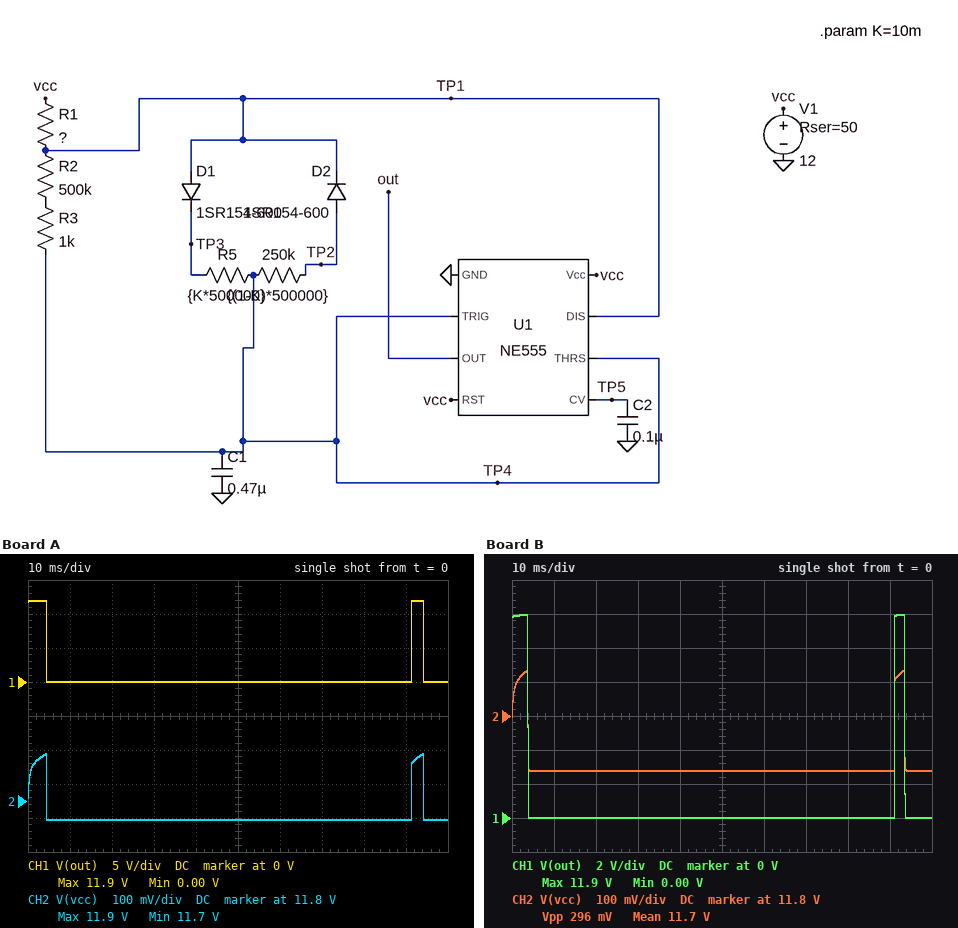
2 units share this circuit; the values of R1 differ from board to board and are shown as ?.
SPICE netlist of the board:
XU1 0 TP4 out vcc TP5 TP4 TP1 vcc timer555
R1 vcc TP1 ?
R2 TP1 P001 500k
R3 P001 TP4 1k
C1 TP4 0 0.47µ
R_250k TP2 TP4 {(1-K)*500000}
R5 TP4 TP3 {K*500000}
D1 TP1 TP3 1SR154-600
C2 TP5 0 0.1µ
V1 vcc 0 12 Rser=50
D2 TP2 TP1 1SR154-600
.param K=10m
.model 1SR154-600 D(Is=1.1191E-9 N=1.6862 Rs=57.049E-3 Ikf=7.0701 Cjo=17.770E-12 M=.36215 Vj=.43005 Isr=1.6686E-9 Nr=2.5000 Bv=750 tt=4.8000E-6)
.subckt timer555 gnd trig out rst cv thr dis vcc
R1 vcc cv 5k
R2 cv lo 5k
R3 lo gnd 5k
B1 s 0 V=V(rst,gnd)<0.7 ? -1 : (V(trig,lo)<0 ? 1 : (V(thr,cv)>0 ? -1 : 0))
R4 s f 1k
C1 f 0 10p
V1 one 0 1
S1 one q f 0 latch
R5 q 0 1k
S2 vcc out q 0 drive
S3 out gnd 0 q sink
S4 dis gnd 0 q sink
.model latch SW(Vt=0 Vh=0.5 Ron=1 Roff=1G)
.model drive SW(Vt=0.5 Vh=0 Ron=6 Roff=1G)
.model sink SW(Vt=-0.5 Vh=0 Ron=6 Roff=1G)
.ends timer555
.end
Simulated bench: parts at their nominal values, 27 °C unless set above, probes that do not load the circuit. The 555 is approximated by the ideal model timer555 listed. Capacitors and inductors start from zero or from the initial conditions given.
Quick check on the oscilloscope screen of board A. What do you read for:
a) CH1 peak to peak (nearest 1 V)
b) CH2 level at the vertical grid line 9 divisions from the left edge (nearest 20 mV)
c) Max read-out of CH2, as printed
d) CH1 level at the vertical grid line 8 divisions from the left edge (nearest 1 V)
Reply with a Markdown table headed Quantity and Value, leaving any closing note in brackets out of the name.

| Quantity | Value |
|---|---|
| CH1 peak to peak | 12 V |
| CH2 level at the vertical grid line 9 divisions from the left edge | 11.74 V |
| Max read-out of CH2, as printed | 11.9 V |
| CH1 level at the vertical grid line 8 divisions from the left edge | 0 V |
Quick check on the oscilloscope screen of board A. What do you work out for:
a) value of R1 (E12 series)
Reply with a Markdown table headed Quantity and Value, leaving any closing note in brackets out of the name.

| Quantity | Value |
|---|---|
| value of R1 | 2.7 kΩ |
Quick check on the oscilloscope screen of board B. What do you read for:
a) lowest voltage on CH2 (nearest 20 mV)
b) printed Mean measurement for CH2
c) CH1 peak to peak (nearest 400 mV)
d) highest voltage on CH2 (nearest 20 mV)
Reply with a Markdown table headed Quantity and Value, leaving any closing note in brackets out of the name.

| Quantity | Value |
|---|---|
| lowest voltage on CH2 | 11.64 V |
| printed Mean measurement for CH2 | 11.7 V |
| CH1 peak to peak | 12.0 V |
| highest voltage on CH2 | 11.94 V |
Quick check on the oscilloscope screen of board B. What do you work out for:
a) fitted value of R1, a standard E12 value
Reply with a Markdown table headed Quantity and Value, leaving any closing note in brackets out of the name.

| Quantity | Value |
|---|---|
| fitted value of R1, a standard E12 value | 1.8 kΩ |
